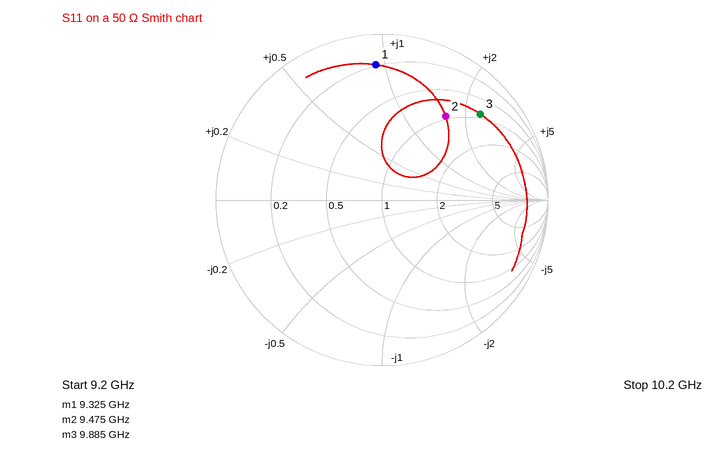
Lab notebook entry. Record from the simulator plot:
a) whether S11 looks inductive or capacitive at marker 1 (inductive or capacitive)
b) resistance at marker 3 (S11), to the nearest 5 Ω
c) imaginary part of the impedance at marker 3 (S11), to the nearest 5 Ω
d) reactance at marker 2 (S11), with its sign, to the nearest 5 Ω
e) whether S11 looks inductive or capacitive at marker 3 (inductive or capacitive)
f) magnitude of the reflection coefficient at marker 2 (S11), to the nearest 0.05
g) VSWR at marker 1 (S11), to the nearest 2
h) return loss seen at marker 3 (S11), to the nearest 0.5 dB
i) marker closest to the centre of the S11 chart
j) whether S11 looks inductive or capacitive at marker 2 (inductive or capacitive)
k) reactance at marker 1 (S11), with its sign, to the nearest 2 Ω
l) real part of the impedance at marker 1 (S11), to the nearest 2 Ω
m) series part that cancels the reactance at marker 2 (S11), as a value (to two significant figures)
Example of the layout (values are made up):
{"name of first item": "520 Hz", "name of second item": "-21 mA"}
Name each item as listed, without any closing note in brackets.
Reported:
{"whether S11 looks inductive or capacitive at marker 1": "inductive", "resistance at marker 3 (S11), to the nearest 5 Ω": "45 Ω", "imaginary part of the impedance at marker 3 (S11), to the nearest 5 Ω": "+120 Ω", "reactance at marker 2 (S11), with its sign, to the nearest 5 Ω": "+80 Ω", "whether S11 looks inductive or capacitive at marker 3": "inductive", "magnitude of the reflection coefficient at marker 2 (S11), to the nearest 0.05": "0.65", "VSWR at marker 1 (S11), to the nearest 2": "10", "return loss seen at marker 3 (S11), to the nearest 0.5 dB": "2.0 dB", "marker closest to the centre of the S11 chart": "marker 2", "whether S11 looks inductive or capacitive at marker 2": "inductive", "reactance at marker 1 (S11), with its sign, to the nearest 2 Ω": "+46 Ω", "real part of the impedance at marker 1 (S11), to the nearest 2 Ω": "10 Ω", "series part that cancels the reactance at marker 2 (S11), as a value": "210 fF"}
